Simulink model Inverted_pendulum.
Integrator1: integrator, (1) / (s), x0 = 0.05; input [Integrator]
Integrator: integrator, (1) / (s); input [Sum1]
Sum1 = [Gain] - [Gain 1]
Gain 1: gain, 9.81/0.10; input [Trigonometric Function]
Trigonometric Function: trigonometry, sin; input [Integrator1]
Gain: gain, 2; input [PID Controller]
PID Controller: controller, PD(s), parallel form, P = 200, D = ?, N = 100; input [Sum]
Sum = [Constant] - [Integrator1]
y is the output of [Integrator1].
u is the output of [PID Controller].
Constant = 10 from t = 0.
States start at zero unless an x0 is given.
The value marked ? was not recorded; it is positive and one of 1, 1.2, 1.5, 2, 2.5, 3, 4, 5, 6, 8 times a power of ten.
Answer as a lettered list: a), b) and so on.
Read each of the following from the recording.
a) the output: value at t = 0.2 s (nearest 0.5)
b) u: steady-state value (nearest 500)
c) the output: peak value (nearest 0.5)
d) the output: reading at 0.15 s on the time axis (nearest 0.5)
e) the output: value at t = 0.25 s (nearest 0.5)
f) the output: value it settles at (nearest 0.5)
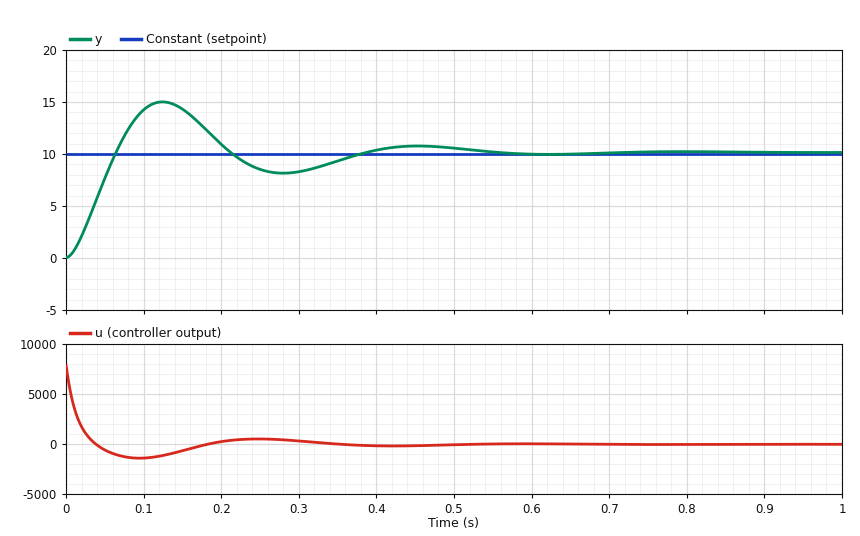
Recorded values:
a) 11.0
b) 0
c) 15.0
d) 14.5
e) 8.5
f) 10.0
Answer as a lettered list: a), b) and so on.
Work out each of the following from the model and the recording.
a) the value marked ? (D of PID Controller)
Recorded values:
a) 6
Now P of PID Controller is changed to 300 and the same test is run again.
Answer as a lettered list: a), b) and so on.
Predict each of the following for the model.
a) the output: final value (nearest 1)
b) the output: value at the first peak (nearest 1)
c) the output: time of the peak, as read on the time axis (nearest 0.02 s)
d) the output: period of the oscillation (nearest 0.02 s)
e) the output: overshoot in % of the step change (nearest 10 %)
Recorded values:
a) 10
b) 16
c) 0.10 s
d) 0.26 s
e) 60 %
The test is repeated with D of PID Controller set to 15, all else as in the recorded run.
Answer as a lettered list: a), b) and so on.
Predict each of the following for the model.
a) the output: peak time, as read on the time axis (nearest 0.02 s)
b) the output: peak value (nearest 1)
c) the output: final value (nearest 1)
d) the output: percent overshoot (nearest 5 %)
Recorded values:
a) 0.08 s
b) 13
c) 10
d) 25 %
